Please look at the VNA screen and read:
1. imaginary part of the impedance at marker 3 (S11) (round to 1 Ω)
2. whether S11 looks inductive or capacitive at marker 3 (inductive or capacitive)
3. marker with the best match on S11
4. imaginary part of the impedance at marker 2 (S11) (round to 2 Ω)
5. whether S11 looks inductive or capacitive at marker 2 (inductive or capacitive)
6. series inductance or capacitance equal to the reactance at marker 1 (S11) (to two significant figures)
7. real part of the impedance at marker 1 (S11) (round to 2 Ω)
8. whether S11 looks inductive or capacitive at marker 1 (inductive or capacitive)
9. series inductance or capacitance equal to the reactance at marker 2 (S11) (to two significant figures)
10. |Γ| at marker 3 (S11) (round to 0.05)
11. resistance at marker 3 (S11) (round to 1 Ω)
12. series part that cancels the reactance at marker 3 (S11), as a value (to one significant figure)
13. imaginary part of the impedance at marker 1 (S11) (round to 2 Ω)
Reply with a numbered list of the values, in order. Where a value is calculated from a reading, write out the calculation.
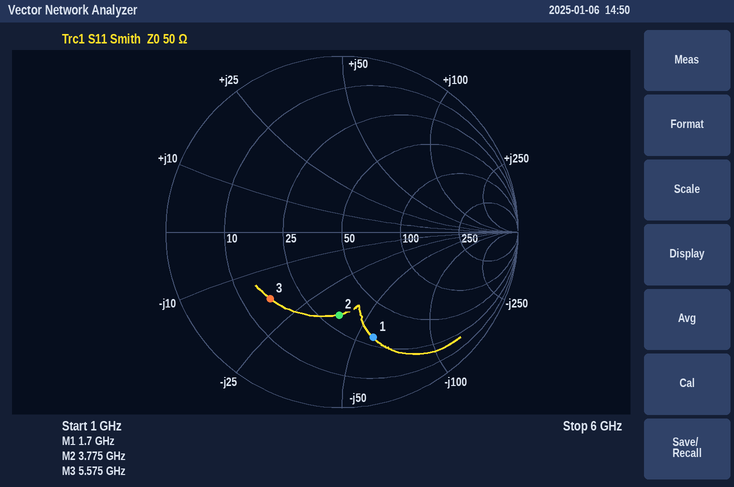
1. -18 Ω
2. capacitive
3. marker 2
4. -38 Ω
5. capacitive
6. C = 1/(2π × 1.7 GHz × 58 Ω) ≈ 1.6 pF
7. 30 Ω
8. capacitive
9. C = 1/(2π × 3.775 GHz × 38 Ω) ≈ 1.1 pF
10. 0.55
11. 16 Ω
12. L = 18 Ω/(2π × 5.575 GHz) ≈ 514 pH, so 500 pH to one significant figure
13. -58 Ω
